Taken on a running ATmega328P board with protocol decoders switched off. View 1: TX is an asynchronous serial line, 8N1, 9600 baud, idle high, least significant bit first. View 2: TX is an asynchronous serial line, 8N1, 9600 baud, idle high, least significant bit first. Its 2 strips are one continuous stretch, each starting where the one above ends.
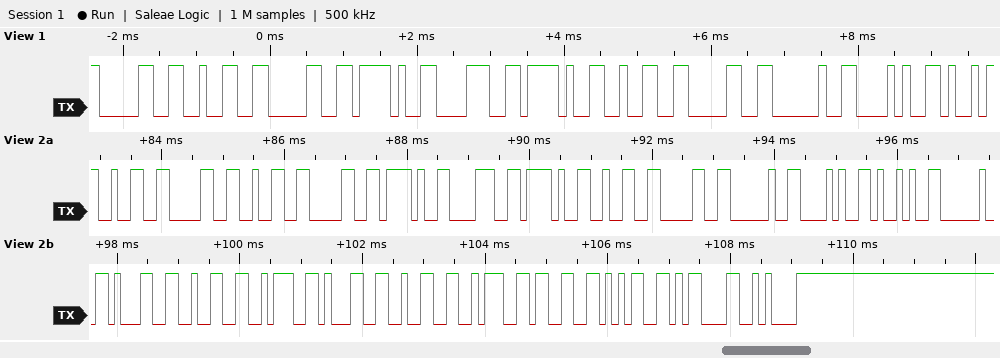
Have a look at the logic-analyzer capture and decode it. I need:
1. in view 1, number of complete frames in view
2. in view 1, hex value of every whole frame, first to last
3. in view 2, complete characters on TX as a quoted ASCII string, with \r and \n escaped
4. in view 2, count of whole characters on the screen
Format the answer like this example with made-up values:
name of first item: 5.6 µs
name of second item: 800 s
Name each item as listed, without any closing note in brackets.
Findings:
in view 1, number of complete frames in view: 10
in view 1, hex value of every whole frame, first to last: 0x30 0x32 0x30 0x2F 0x38 0x2F 0x32 0x30 0x20 0x28
in view 2, complete characters on TX as a quoted ASCII string, with \r and \n escaped: "2020/8/20 () 12:12:35\r\n"
in view 2, count of whole characters on the screen: 23
